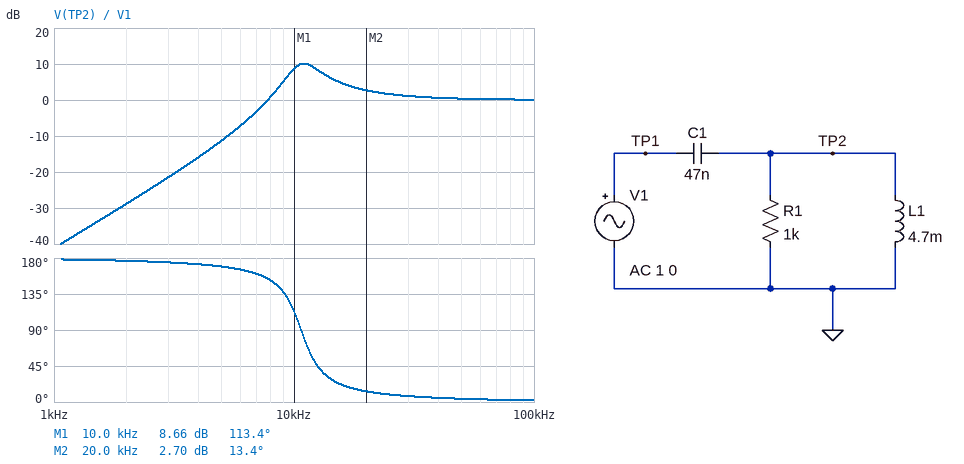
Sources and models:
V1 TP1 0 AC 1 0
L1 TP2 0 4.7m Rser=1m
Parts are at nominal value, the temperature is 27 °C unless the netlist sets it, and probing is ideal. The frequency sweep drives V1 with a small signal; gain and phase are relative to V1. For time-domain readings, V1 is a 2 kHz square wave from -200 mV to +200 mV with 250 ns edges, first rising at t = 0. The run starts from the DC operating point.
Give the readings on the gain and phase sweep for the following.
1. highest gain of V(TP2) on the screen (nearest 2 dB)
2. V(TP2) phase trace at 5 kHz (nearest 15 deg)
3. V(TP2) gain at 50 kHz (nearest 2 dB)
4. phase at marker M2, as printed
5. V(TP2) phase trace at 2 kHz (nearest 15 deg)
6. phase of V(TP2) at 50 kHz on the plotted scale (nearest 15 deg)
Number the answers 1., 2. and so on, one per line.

1. 10 dB
2. 165 deg
3. 0 dB
4. 13.4 deg
5. 180 deg
6. 0 deg
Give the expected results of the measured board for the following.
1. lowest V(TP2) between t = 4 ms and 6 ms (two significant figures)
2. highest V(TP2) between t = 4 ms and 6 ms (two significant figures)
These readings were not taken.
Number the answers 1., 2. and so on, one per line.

1. -410 mV
2. 410 mV
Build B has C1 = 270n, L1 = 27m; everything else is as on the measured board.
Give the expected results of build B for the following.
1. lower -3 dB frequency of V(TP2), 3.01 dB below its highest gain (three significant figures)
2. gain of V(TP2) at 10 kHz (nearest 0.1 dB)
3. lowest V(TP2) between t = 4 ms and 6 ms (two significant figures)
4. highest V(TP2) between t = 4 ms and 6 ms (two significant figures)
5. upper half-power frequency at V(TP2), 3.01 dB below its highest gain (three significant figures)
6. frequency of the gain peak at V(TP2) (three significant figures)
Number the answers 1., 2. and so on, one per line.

1. 1.66 kHz
2. 0.3 dB
3. -940 mV
4. 940 mV
5. 2.33 kHz
6. 1.91 kHz
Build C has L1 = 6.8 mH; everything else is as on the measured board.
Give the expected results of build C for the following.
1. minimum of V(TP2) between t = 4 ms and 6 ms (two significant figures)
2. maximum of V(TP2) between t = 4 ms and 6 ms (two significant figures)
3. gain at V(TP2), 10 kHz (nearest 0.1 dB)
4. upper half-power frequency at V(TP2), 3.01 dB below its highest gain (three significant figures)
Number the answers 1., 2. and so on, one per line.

1. -390 mV
2. 390 mV
3. 8.0 dB
4. 12.0 kHz
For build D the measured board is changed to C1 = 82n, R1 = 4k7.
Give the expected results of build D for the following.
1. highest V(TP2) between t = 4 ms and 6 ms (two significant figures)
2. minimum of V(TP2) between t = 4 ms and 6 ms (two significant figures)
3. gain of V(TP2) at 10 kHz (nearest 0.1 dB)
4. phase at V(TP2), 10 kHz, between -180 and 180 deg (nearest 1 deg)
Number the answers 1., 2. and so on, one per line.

1. 230 mV
2. -230 mV
3. 9.2 dB
4. 7 deg
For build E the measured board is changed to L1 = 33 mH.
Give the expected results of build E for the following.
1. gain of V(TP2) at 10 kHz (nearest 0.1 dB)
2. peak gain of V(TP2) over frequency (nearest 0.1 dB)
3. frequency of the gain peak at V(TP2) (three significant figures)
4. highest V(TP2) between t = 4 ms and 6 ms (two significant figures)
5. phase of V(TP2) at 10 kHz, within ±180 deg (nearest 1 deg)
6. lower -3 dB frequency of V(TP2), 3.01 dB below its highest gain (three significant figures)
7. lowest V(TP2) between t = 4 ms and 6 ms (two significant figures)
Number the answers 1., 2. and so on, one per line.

1. 0.9 dB
2. 2.4 dB
3. 5.02 kHz
4. 370 mV
5. 22 deg
6. 3.40 kHz
7. -370 mV
